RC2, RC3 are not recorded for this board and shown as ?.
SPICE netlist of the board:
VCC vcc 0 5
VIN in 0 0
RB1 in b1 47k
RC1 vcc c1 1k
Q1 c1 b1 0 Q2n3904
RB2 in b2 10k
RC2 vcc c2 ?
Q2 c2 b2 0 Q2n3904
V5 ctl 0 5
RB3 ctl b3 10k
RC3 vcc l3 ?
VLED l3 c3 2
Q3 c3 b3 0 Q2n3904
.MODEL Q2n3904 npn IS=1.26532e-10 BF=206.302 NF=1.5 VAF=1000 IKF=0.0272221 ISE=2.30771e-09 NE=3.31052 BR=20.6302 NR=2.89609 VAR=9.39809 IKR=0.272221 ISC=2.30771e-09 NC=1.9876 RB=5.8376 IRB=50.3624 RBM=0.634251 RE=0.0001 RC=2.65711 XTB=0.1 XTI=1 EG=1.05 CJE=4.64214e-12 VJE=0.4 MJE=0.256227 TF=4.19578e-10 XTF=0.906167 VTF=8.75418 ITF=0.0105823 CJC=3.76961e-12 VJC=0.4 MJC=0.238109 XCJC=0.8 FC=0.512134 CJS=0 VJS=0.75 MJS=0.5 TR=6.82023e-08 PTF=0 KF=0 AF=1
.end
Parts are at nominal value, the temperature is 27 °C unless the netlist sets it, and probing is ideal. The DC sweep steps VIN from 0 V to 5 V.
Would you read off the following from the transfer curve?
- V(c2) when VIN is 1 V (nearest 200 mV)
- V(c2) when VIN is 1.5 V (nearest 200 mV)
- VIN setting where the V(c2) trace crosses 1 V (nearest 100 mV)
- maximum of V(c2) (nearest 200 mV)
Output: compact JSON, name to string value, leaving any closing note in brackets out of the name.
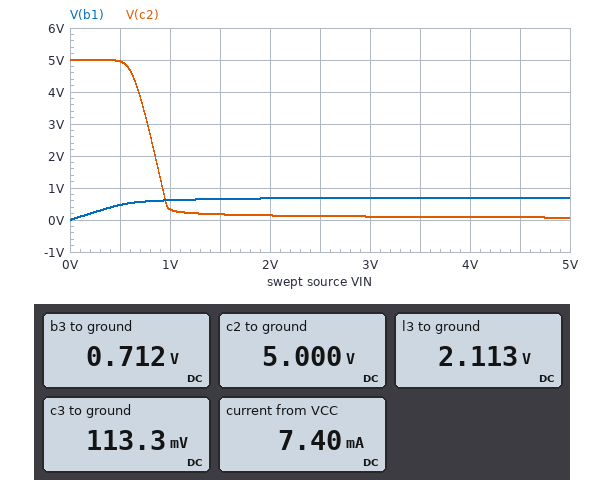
{"V(c2) when VIN is 1 V": "400 mV", "V(c2) when VIN is 1.5 V": "200 mV", "VIN setting where the V(c2) trace crosses 1 V": "900 mV", "maximum of V(c2)": "5.0 V"}
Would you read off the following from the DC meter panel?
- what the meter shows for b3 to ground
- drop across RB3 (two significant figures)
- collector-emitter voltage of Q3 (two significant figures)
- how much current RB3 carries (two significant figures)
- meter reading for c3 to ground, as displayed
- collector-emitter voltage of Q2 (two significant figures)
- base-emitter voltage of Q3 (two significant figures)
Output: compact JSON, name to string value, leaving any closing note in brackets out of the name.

{"what the meter shows for b3 to ground": "0.712 V", "drop across RB3": "4.3 V", "collector-emitter voltage of Q3": "110 mV", "how much current RB3 carries": "430 µA", "meter reading for c3 to ground, as displayed": "113.3 mV", "collector-emitter voltage of Q2": "5.0 V", "base-emitter voltage of Q3": "710 mV"}
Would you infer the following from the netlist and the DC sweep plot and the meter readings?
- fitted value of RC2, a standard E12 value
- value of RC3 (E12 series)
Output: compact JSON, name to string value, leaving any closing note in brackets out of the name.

{"fitted value of RC2, a standard E12 value": "1.2 kΩ", "value of RC3": "390 Ω"}
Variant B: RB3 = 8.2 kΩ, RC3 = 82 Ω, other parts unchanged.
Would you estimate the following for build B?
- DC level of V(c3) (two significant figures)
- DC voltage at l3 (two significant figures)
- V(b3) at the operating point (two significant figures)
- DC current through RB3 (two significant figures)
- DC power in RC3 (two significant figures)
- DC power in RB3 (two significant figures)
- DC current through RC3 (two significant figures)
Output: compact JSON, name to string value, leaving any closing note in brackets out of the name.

{"DC level of V(c3)": "330 mV", "DC voltage at l3": "2.3 V", "V(b3) at the operating point": "790 mV", "DC current through RB3": "510 µA", "DC power in RC3": "87 mW", "DC power in RB3": "2.2 mW", "DC current through RC3": "33 mA"}
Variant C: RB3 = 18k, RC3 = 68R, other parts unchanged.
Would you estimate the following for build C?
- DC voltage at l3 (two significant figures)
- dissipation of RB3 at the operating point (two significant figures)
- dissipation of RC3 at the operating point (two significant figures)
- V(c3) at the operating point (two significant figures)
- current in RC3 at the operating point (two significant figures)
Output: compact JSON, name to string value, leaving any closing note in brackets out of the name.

{"DC voltage at l3": "3.5 V", "dissipation of RB3 at the operating point": "1.0 mW", "dissipation of RC3 at the operating point": "33 mW", "V(c3) at the operating point": "1.5 V", "current in RC3 at the operating point": "22 mA"}
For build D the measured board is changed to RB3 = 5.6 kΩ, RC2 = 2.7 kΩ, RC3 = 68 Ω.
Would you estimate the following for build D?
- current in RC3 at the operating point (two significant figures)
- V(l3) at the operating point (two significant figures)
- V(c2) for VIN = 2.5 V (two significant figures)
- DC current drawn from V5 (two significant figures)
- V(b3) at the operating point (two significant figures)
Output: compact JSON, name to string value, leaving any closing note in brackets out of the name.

{"current in RC3 at the operating point": "39 mA", "V(l3) at the operating point": "2.3 V", "V(c2) for VIN = 2.5 V": "78 mV", "DC current drawn from V5": "750 µA", "V(b3) at the operating point": "800 mV"}
